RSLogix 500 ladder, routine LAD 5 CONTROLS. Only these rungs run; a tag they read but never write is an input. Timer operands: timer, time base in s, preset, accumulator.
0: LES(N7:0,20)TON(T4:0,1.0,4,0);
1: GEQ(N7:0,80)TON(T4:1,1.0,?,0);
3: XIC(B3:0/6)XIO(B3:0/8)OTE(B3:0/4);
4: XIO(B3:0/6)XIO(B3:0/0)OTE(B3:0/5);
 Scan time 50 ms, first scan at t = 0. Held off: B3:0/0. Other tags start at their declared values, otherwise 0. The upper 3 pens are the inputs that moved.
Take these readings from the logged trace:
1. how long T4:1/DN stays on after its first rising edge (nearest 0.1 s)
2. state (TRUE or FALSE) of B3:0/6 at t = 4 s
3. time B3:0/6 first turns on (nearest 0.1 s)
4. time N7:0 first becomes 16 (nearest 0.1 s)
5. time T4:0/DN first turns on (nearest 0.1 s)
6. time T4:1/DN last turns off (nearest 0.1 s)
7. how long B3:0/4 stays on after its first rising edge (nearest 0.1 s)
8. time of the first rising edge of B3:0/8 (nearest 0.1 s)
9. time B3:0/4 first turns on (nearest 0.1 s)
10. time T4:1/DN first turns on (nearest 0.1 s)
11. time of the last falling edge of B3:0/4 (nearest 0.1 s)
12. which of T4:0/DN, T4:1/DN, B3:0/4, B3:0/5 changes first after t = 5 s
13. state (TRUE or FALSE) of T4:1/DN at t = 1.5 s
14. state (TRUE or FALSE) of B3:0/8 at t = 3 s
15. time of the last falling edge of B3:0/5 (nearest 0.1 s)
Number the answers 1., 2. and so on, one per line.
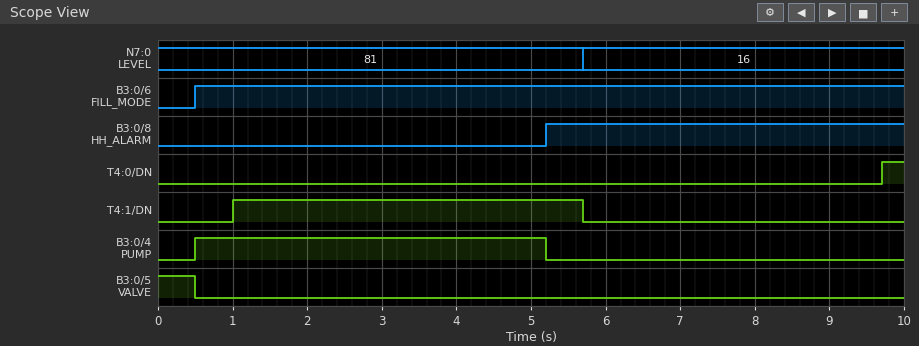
1. 4.7 s
2. TRUE
3. 0.5 s
4. 5.7 s
5. 9.7 s
6. 5.7 s
7. 4.7 s
8. 5.2 s
9. 0.5 s
10. 1.0 s
11. 5.2 s
12. B3:0/4
13. TRUE
14. FALSE
15. 0.5 s
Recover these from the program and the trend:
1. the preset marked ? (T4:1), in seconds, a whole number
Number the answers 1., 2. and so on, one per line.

1. 1 s
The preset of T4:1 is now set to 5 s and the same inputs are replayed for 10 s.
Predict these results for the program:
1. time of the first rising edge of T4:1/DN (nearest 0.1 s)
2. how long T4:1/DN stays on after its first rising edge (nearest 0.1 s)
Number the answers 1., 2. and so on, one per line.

1. 5.0 s
2. 0.7 s
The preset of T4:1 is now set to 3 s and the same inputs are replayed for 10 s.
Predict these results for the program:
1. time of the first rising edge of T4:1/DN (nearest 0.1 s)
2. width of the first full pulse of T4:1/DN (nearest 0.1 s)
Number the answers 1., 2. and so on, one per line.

1. 3.0 s
2. 2.7 s
